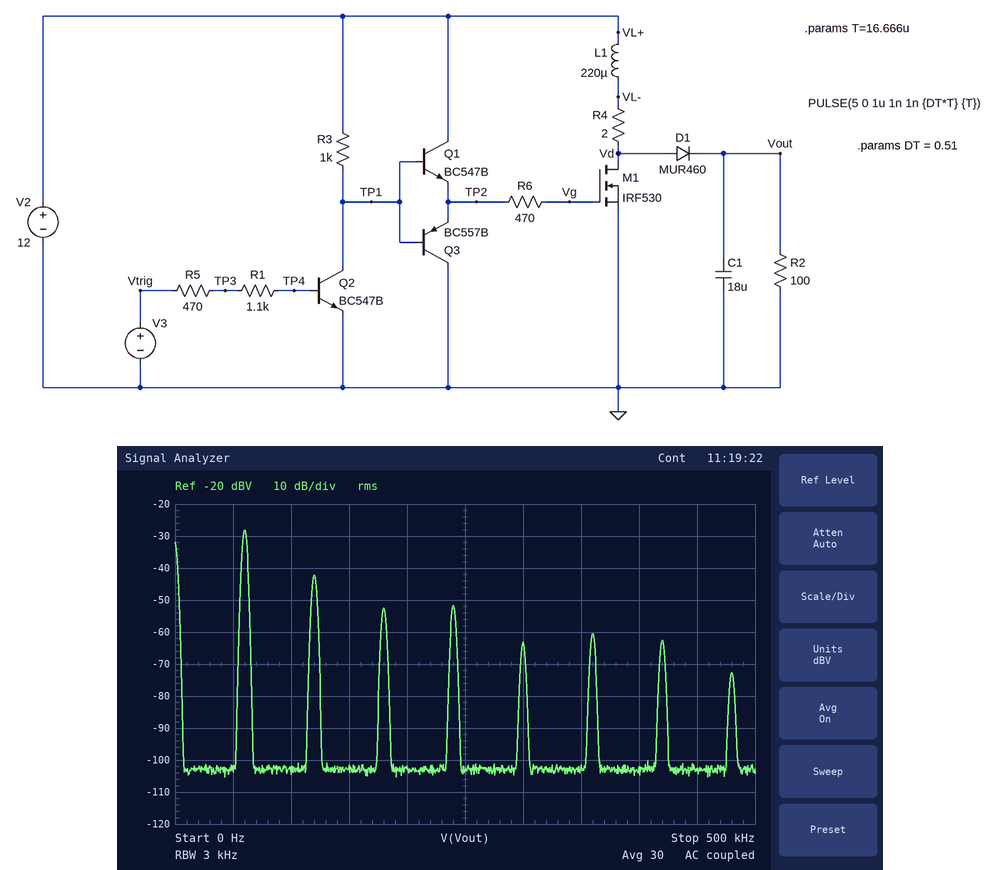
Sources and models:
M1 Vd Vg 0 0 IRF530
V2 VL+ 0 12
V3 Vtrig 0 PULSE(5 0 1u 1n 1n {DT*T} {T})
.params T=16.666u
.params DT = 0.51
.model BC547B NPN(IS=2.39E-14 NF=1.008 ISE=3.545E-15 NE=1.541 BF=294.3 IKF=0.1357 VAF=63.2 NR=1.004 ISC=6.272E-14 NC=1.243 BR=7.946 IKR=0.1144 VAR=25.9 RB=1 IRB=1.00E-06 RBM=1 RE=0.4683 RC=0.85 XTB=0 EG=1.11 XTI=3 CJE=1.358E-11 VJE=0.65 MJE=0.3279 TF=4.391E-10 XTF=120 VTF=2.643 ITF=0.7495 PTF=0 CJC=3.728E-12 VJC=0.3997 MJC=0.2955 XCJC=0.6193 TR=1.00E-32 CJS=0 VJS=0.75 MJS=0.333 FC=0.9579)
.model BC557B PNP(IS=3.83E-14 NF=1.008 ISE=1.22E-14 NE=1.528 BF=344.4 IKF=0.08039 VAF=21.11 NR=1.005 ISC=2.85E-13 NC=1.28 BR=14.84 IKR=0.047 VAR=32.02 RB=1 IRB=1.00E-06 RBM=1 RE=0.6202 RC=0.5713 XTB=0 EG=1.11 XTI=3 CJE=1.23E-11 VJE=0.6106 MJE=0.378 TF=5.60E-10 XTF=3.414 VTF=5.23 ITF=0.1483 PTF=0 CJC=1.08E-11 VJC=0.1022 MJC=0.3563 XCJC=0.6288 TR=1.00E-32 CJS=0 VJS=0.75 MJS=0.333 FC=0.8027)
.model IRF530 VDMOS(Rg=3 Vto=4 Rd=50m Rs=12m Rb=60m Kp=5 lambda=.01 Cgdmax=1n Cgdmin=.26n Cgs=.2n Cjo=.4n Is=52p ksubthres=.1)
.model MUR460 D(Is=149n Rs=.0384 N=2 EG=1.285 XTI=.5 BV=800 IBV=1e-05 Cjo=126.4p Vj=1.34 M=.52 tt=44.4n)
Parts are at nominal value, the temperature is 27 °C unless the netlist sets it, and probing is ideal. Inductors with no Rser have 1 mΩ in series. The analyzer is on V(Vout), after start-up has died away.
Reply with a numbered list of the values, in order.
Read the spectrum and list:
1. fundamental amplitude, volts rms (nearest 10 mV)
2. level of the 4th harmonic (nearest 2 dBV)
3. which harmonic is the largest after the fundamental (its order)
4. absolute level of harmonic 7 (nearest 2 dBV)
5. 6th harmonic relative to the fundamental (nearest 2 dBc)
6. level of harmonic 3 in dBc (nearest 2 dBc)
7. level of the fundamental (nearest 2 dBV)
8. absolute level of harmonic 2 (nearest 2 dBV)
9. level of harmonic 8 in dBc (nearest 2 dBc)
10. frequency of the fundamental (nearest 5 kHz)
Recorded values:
1. 40 mV
2. -52 dBV
3. 2
4. -62 dBV
5. -32 dBc
6. -24 dBc
7. -28 dBV
8. -42 dBV
9. -44 dBc
10. 60 kHz
